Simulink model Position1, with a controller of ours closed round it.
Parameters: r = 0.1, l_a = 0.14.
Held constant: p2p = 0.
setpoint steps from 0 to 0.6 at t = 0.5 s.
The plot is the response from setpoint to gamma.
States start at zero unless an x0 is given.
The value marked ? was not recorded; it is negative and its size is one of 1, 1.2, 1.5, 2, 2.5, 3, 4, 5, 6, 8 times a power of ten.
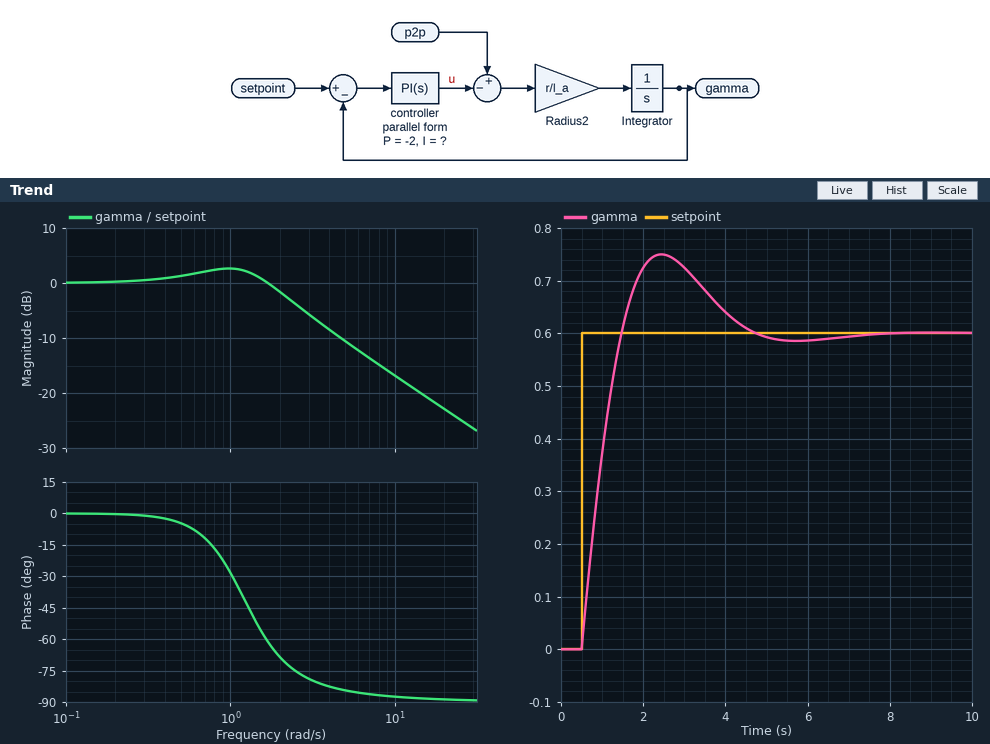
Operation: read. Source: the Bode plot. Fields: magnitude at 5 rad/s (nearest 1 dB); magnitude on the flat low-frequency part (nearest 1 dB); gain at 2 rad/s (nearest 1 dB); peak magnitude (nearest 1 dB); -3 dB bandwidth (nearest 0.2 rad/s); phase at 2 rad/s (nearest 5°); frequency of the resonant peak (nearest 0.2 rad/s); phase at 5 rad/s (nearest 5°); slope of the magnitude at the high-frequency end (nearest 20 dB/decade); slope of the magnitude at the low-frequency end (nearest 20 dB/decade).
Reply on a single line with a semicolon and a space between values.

-11 dB; 0 dB; -2 dB; 3 dB; 2.2 rad/s; -70°; 1.0 rad/s; -85°; -20 dB/decade; 0 dB/decade
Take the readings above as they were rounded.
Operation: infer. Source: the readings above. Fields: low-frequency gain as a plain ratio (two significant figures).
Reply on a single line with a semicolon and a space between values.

1.0
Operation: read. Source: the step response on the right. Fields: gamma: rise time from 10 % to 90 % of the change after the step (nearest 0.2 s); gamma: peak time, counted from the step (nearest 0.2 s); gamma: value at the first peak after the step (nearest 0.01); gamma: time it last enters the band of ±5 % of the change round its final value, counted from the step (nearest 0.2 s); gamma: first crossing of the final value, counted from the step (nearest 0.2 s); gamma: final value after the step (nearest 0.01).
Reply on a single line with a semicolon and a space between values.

0.8 s; 2.0 s; 0.75; 3.6 s; 1.0 s; 0.60
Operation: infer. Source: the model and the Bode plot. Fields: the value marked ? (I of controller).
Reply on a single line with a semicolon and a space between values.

-2
